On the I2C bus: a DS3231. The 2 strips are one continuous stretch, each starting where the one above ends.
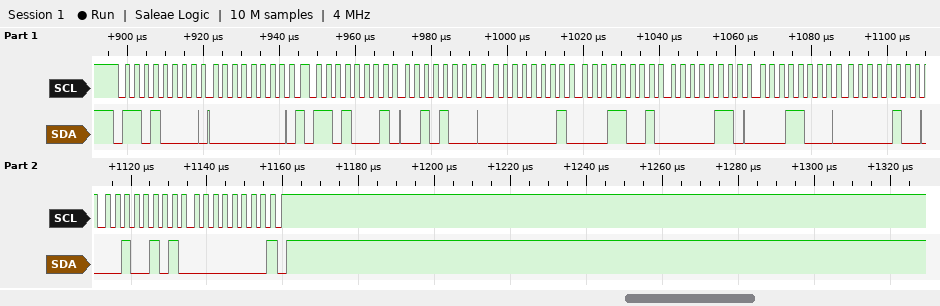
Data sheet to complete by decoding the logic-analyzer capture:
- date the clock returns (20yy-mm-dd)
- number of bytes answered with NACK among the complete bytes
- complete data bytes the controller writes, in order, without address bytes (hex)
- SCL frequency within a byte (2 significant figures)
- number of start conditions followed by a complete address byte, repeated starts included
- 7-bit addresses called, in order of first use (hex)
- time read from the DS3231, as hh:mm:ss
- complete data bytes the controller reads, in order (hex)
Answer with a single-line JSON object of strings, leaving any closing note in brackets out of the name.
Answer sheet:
{"date the clock returns": "2025-04-18", "number of bytes answered with NACK among the complete bytes": "1", "complete data bytes the controller writes, in order, without address bytes": "00", "SCL frequency within a byte": "400 kHz", "number of start conditions followed by a complete address byte, repeated starts included": "2", "7-bit addresses called, in order of first use": "0x68", "time read from the DS3231, as hh:mm:ss": "19:01:28", "complete data bytes the controller reads, in order": "28 01 19 06 18 04 25 00"}
